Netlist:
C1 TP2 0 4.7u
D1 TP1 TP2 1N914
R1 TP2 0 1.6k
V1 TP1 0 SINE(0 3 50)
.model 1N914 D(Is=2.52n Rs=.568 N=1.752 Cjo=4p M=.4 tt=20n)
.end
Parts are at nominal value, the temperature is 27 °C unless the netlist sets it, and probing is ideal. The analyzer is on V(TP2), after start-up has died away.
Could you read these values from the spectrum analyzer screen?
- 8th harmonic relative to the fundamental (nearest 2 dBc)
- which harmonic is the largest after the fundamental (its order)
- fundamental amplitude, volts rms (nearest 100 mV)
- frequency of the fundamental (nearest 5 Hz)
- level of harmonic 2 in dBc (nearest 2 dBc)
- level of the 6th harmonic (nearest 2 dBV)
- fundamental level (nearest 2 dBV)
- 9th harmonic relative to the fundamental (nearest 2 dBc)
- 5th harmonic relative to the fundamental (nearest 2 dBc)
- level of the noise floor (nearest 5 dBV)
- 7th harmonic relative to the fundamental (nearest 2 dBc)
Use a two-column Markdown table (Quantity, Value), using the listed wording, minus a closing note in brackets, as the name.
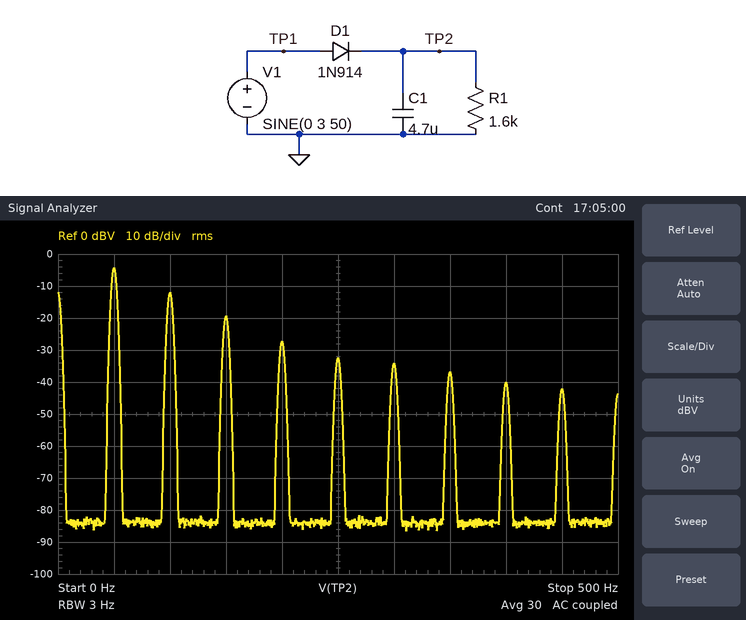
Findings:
| Quantity | Value |
|---|---|
| 8th harmonic relative to the fundamental | -36 dBc |
| which harmonic is the largest after the fundamental | 2 |
| fundamental amplitude, volts rms | 600 mV |
| frequency of the fundamental | 50 Hz |
| level of harmonic 2 in dBc | -8 dBc |
| level of the 6th harmonic | -34 dBV |
| fundamental level | -4 dBV |
| 9th harmonic relative to the fundamental | -38 dBc |
| 5th harmonic relative to the fundamental | -28 dBc |
| level of the noise floor | -85 dBV |
| 7th harmonic relative to the fundamental | -32 dBc |
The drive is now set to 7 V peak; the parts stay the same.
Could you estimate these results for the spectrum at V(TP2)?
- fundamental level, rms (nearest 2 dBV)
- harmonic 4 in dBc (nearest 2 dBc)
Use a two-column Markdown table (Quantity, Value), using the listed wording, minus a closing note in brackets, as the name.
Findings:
| Quantity | Value |
|---|---|
| fundamental level, rms | 4 dBV |
| harmonic 4 in dBc | -24 dBc |
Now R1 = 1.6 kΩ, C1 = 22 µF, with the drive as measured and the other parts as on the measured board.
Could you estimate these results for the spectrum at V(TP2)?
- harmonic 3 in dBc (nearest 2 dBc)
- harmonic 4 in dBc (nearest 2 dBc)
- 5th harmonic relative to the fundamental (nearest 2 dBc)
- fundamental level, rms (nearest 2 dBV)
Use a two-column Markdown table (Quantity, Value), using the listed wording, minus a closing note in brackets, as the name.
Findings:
| Quantity | Value |
|---|---|
| harmonic 3 in dBc | -12 dBc |
| harmonic 4 in dBc | -16 dBc |
| 5th harmonic relative to the fundamental | -20 dBc |
| fundamental level, rms | -12 dBV |
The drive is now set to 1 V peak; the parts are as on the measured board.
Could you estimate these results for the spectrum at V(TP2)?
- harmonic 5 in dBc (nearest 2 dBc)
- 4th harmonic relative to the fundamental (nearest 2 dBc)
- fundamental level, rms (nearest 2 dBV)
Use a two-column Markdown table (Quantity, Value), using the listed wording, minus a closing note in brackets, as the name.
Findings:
| Quantity | Value |
|---|---|
| harmonic 5 in dBc | -24 dBc |
| 4th harmonic relative to the fundamental | -18 dBc |
| fundamental level, rms | -18 dBV |
